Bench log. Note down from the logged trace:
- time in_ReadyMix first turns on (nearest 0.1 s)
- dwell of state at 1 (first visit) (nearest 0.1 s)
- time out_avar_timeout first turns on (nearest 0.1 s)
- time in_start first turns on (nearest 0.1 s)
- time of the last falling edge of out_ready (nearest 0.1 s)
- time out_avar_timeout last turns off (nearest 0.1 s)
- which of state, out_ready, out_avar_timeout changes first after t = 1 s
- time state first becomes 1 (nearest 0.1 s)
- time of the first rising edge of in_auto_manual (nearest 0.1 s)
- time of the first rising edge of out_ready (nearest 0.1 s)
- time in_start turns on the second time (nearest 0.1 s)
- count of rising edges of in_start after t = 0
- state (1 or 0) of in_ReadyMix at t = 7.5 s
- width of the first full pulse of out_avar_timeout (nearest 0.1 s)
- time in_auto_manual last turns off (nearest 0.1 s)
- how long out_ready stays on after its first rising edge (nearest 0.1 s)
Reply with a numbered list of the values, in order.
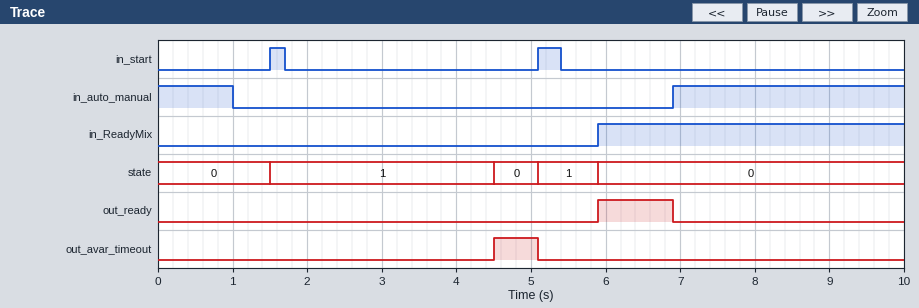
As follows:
1. 5.9 s
2. 3.0 s
3. 4.5 s
4. 1.5 s
5. 6.9 s
6. 5.1 s
7. state
8. 1.5 s
9. 6.9 s
10. 5.9 s
11. 5.1 s
12. 2
13. 1
14. 0.6 s
15. 1.0 s
16. 1.0 s
